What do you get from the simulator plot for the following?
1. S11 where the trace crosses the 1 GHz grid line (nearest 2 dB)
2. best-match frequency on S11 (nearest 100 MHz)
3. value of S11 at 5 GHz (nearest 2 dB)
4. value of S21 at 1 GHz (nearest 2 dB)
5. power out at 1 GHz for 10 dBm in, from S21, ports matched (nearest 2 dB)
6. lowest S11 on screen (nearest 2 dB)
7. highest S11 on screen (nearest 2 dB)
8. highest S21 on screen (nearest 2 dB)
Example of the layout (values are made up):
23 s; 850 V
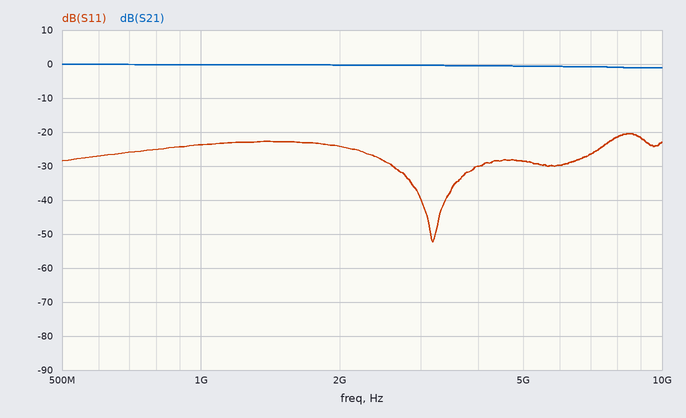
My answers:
-24 dB; 3.2 GHz; -28 dB; 0 dB; 10 dBm; -52 dB; -20 dB; 0 dB
